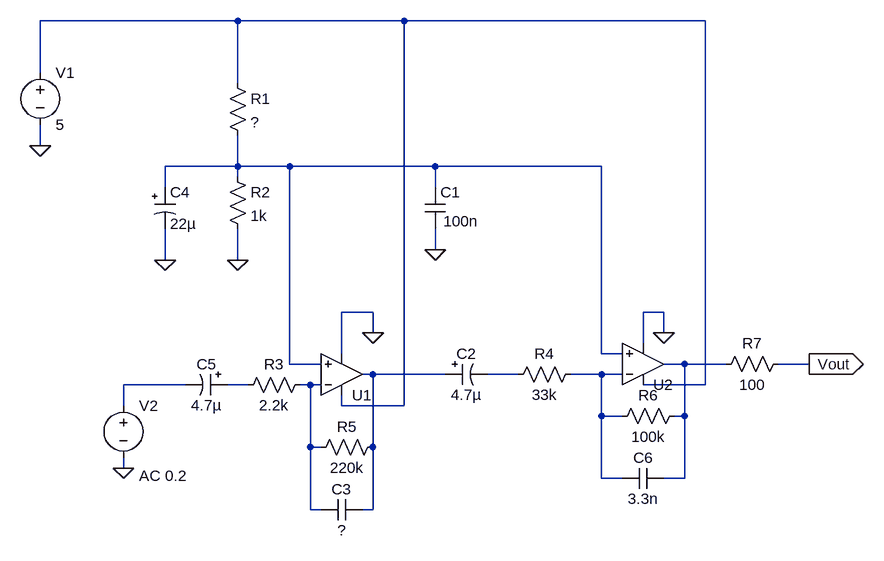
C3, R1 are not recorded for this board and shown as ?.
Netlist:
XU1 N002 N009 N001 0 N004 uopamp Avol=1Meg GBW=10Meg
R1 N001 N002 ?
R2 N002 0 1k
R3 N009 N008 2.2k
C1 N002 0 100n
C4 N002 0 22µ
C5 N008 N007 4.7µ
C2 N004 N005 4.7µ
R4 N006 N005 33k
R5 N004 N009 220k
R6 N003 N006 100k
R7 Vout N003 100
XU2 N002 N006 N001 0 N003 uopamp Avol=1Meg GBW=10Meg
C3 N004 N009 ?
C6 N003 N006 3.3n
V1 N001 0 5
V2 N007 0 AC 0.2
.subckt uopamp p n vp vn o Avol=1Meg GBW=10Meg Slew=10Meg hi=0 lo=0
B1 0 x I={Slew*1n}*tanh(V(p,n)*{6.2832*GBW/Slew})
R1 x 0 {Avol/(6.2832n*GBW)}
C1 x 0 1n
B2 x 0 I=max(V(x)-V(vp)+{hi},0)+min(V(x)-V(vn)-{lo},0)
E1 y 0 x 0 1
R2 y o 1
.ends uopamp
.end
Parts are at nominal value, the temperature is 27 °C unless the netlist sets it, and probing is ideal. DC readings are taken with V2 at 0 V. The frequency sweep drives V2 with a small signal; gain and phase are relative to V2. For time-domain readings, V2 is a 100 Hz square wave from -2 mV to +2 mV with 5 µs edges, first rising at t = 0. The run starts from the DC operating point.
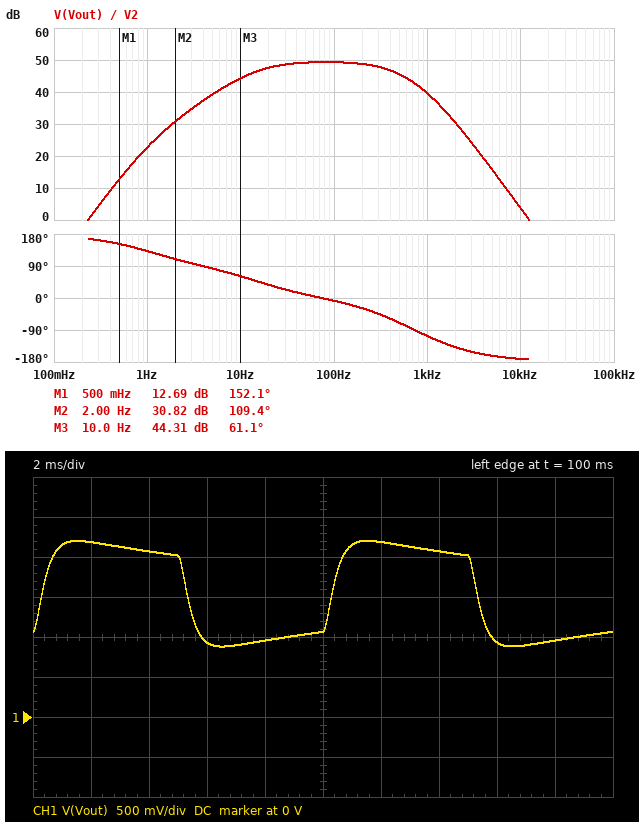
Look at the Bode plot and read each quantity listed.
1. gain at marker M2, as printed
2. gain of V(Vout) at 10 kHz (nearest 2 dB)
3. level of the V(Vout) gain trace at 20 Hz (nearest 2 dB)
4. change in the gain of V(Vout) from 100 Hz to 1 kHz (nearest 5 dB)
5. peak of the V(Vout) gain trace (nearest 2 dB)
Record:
30.82 dB
4 dB
48 dB
-10 dB
50 dB
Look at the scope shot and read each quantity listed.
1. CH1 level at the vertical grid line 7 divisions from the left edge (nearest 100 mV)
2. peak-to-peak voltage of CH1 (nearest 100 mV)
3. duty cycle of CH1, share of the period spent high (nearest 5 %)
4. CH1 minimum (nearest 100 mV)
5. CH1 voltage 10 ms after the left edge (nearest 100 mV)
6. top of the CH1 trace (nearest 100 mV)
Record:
2.1 V
1.3 V
50 %
900 mV
1.1 V
2.2 V
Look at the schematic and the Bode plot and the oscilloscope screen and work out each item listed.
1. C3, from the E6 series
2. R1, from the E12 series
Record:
680 pF
2.2 kΩ
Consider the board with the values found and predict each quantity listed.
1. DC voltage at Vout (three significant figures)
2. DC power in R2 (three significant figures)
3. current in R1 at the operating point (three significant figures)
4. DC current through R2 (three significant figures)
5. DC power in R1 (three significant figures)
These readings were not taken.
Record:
1.56 V
2.44 mW
1.56 mA
1.56 mA
5.37 mW
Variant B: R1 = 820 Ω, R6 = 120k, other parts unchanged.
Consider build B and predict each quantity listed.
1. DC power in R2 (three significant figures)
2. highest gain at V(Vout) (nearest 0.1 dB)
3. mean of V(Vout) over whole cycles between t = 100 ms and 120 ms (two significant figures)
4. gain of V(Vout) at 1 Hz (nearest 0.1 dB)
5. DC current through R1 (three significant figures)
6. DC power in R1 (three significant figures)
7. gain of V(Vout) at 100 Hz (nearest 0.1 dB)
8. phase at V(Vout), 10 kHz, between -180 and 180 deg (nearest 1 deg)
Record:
7.55 mW
50.9 dB
2.7 V
24.3 dB
2.75 mA
6.19 mW
50.8 dB
-172 deg
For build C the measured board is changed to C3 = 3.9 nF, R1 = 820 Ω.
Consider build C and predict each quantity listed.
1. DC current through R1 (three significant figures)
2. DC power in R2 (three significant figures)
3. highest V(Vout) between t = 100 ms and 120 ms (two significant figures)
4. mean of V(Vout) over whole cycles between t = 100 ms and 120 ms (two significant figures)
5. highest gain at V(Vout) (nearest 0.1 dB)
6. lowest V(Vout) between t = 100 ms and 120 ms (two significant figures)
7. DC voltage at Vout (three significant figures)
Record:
2.75 mA
7.55 mW
3.3 V
2.7 V
48.9 dB
2.2 V
2.75 V
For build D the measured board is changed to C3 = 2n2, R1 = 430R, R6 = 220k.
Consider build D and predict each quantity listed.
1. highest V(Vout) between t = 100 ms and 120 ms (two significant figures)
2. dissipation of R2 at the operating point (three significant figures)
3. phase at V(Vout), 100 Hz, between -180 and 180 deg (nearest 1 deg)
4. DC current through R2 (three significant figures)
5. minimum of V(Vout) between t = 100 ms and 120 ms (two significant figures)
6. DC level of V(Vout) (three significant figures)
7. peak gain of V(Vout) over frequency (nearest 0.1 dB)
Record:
4.7 V
12.2 mW
-32 deg
3.50 mA
2.2 V
3.50 V
55.8 dB
